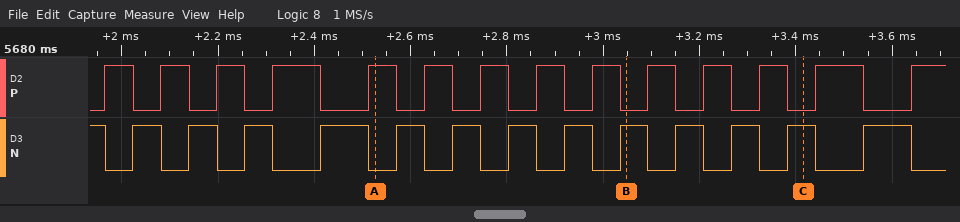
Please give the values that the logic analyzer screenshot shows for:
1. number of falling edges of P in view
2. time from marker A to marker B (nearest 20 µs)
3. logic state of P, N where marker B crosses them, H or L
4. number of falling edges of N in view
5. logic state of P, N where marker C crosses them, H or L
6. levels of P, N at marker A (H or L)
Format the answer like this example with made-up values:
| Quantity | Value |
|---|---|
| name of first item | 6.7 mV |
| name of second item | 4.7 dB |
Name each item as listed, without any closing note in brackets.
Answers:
| Quantity | Value |
|---|---|
| number of falling edges of P in view | 13 |
| time from marker A to marker B | 520 µs |
| logic state of P, N where marker B crosses them, H or L | P=L, N=H |
| number of falling edges of N in view | 14 |
| logic state of P, N where marker C crosses them, H or L | P=L, N=H |
| levels of P, N at marker A | P=H, N=L |
